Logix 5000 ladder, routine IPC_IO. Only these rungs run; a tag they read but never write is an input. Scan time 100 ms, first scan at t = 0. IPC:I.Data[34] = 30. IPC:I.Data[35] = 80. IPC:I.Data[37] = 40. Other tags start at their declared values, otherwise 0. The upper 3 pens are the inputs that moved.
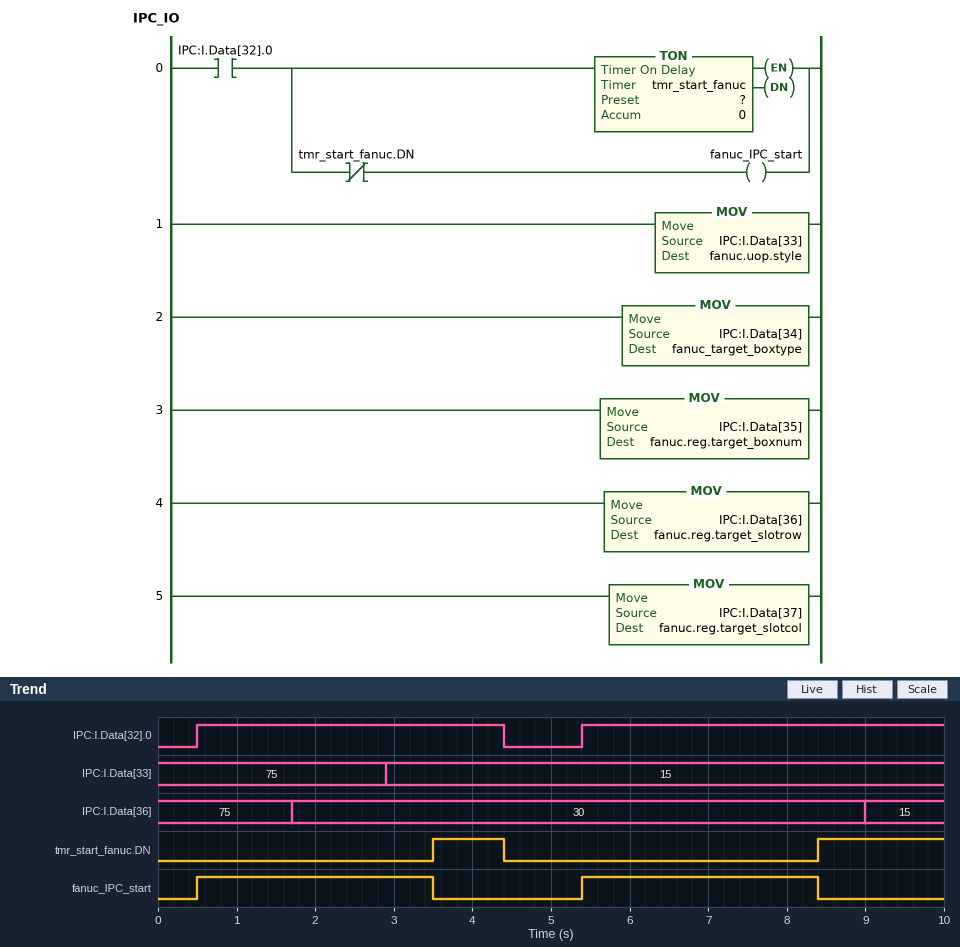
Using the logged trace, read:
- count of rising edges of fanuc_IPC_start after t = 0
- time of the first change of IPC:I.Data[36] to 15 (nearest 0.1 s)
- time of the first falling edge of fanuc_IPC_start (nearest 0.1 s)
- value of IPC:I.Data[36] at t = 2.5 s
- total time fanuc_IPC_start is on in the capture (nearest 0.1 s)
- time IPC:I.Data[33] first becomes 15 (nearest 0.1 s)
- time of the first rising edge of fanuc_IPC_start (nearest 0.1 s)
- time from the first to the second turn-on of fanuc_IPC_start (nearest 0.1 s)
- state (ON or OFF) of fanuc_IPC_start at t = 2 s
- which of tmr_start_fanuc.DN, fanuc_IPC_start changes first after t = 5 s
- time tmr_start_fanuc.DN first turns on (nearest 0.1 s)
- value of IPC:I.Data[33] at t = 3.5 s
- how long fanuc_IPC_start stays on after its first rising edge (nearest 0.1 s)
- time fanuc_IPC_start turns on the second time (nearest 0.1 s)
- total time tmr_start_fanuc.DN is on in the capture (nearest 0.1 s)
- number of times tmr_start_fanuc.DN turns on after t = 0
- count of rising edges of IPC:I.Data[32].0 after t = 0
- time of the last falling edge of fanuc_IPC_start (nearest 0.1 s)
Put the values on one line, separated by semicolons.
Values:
2; 9.0 s; 3.5 s; 30; 6.0 s; 2.9 s; 0.5 s; 4.9 s; ON; fanuc_IPC_start; 3.5 s; 15; 3.0 s; 5.4 s; 2.5 s; 2; 2; 8.4 s
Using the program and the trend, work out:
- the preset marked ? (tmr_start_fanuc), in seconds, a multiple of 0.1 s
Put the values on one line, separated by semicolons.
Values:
3.0 s
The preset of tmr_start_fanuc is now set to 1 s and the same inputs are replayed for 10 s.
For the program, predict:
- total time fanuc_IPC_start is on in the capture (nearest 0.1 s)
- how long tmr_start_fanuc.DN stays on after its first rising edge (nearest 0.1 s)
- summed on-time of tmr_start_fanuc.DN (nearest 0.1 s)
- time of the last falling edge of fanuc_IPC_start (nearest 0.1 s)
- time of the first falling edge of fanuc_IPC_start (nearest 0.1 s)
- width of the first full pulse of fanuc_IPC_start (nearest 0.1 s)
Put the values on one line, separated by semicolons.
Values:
2.0 s; 2.9 s; 6.5 s; 6.4 s; 1.5 s; 1.0 s
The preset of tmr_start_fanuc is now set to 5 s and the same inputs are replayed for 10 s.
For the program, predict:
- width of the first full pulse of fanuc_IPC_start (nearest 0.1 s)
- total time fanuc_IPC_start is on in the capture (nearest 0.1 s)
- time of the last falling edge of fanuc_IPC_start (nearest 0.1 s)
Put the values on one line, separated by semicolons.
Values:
3.9 s; 8.5 s; 4.4 s
